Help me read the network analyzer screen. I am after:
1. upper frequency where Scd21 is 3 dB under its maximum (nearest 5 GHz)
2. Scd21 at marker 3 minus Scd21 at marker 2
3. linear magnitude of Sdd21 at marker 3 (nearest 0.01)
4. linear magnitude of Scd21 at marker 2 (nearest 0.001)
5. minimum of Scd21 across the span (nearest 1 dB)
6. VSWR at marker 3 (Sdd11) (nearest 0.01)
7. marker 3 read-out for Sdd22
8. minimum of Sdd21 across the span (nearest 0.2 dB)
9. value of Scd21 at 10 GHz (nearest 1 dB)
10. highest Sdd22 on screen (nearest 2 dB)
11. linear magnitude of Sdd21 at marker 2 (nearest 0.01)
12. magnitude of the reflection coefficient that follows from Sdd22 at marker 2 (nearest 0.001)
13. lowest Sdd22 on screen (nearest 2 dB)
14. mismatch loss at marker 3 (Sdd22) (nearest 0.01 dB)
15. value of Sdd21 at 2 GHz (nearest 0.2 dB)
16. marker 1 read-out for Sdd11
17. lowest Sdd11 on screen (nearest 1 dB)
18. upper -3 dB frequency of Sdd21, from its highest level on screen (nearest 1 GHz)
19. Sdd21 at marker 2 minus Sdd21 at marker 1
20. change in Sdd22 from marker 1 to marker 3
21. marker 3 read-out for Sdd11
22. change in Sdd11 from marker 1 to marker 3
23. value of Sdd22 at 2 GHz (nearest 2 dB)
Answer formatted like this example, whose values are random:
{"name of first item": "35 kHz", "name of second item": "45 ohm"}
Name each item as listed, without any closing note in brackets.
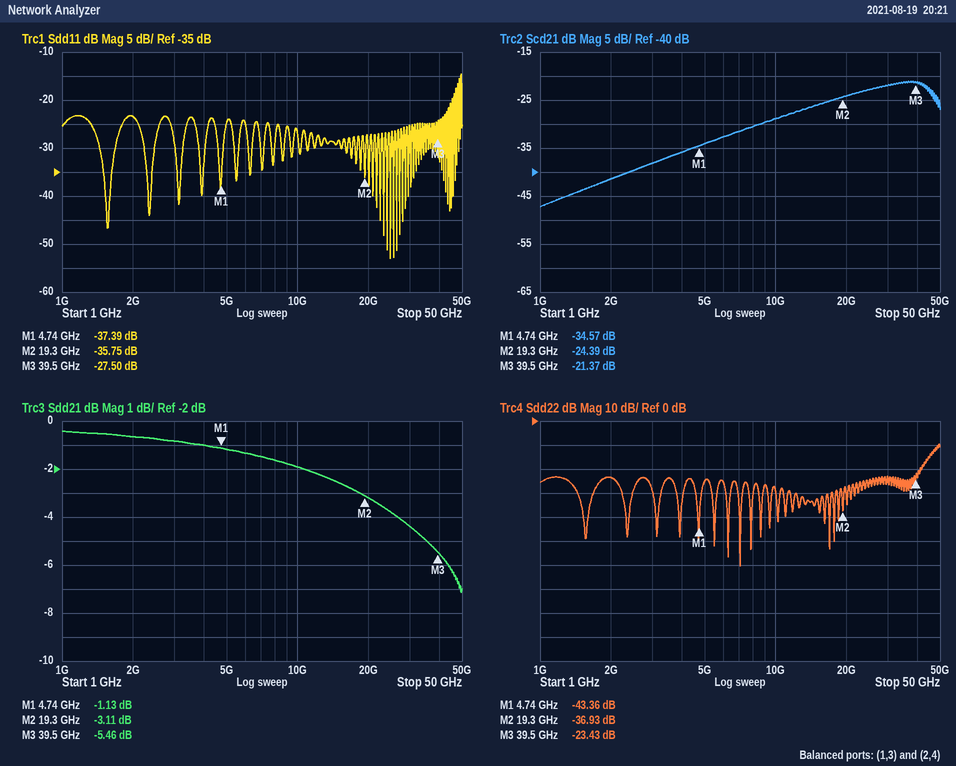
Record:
{"upper frequency where Scd21 is 3 dB under its maximum": "45 GHz", "Scd21 at marker 3 minus Scd21 at marker 2": "3.02 dB", "linear magnitude of Sdd21 at marker 3": "0.53", "linear magnitude of Scd21 at marker 2": "0.060", "minimum of Scd21 across the span": "-47 dB", "VSWR at marker 3 (Sdd11)": "1.09", "marker 3 read-out for Sdd22": "-23.43 dB", "minimum of Sdd21 across the span": "-7.2 dB", "value of Scd21 at 10 GHz": "-29 dB", "highest Sdd22 on screen": "-10 dB", "linear magnitude of Sdd21 at marker 2": "0.70", "magnitude of the reflection coefficient that follows from Sdd22 at marker 2": "0.014", "lowest Sdd22 on screen": "-60 dB", "mismatch loss at marker 3 (Sdd22)": "0.02 dB", "value of Sdd21 at 2 GHz": "-0.6 dB", "marker 1 read-out for Sdd11": "-37.39 dB", "lowest Sdd11 on screen": "-53 dB", "upper -3 dB frequency of Sdd21, from its highest level on screen": "22 GHz", "Sdd21 at marker 2 minus Sdd21 at marker 1": "-1.98 dB", "change in Sdd22 from marker 1 to marker 3": "19.93 dB", "marker 3 read-out for Sdd11": "-27.50 dB", "change in Sdd11 from marker 1 to marker 3": "9.89 dB", "value of Sdd22 at 2 GHz": "-24 dB"}
